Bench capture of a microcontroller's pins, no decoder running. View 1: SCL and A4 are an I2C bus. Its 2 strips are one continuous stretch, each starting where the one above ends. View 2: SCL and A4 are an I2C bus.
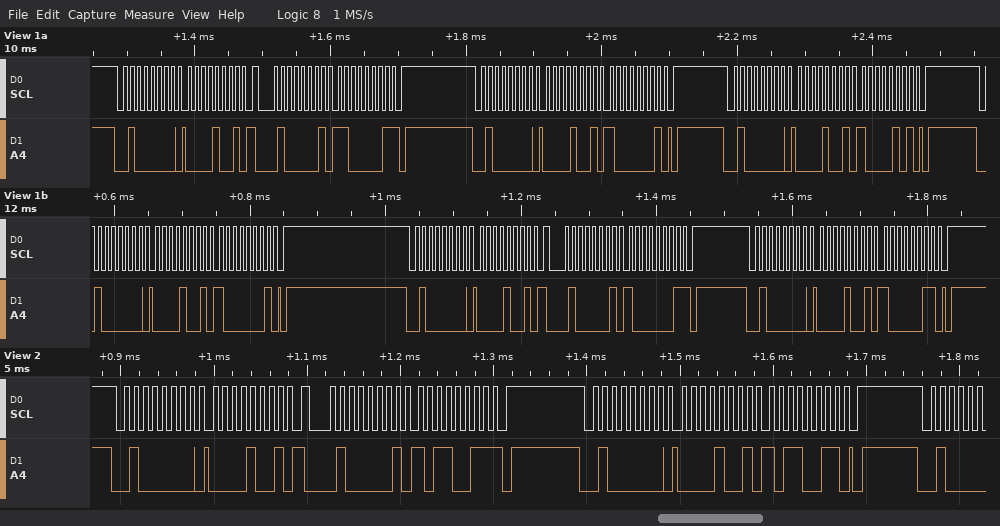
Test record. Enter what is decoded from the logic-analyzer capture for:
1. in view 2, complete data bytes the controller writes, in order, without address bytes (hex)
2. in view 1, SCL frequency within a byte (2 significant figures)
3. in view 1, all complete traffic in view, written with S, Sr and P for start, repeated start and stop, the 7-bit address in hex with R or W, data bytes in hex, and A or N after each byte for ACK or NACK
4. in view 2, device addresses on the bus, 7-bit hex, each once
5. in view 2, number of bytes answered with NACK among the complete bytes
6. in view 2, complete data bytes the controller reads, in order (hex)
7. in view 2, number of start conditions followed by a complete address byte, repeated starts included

09 09 B3
100 kHz
S 20W A 09 A Sr 20R A C1 N P S 20W A 09 A 81 A P S 20W A 09 A 85 A P S 20W A 09 A 81 A P S 20W A 09 A Sr 20R A 81 N P S 20W A 09 A 83 A P
0x20
1
B3
3
